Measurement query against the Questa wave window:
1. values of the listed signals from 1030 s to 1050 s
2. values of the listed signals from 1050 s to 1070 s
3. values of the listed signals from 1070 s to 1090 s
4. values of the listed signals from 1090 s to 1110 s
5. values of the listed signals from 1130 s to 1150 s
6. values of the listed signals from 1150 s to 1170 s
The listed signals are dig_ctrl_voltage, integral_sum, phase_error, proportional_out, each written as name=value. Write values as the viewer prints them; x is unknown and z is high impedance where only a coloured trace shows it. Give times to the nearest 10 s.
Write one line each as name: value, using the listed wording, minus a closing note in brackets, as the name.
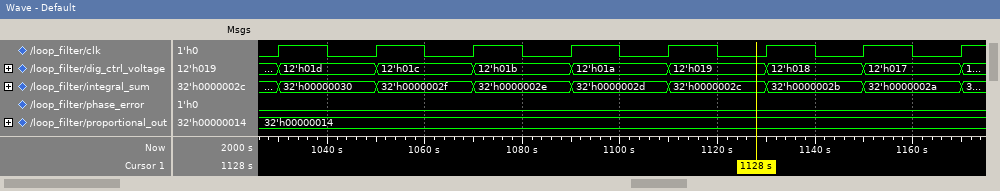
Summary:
values of the listed signals from 1030 s to 1050 s: dig_ctrl_voltage=12'h01d, integral_sum=32'h00000030, phase_error=0, proportional_out=32'h00000014
values of the listed signals from 1050 s to 1070 s: dig_ctrl_voltage=12'h01c, integral_sum=32'h0000002f, phase_error=0, proportional_out=32'h00000014
values of the listed signals from 1070 s to 1090 s: dig_ctrl_voltage=12'h01b, integral_sum=32'h0000002e, phase_error=0, proportional_out=32'h00000014
values of the listed signals from 1090 s to 1110 s: dig_ctrl_voltage=12'h01a, integral_sum=32'h0000002d, phase_error=0, proportional_out=32'h00000014
values of the listed signals from 1130 s to 1150 s: dig_ctrl_voltage=12'h018, integral_sum=32'h0000002b, phase_error=0, proportional_out=32'h00000014
values of the listed signals from 1150 s to 1170 s: dig_ctrl_voltage=12'h017, integral_sum=32'h0000002a, phase_error=0, proportional_out=32'h00000014
